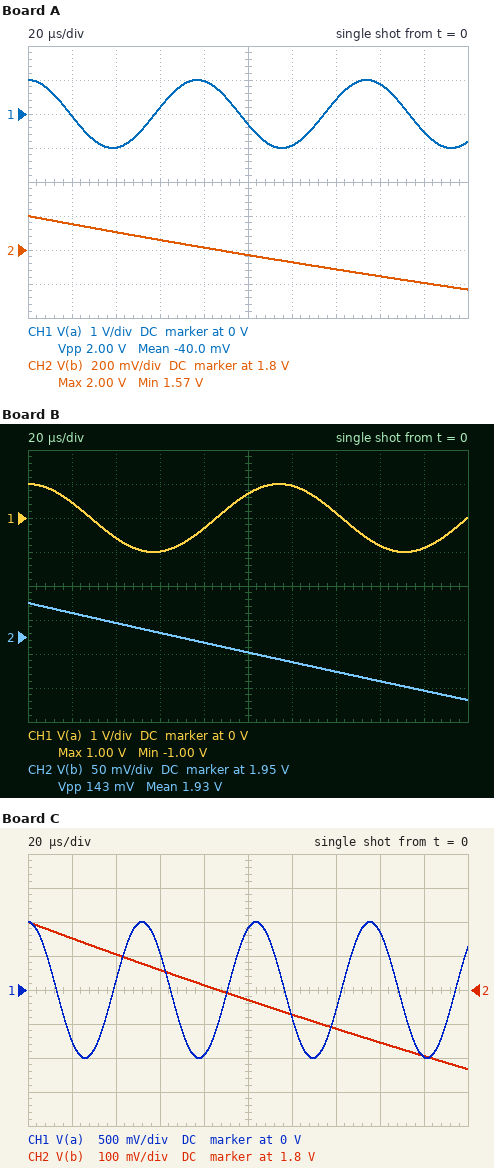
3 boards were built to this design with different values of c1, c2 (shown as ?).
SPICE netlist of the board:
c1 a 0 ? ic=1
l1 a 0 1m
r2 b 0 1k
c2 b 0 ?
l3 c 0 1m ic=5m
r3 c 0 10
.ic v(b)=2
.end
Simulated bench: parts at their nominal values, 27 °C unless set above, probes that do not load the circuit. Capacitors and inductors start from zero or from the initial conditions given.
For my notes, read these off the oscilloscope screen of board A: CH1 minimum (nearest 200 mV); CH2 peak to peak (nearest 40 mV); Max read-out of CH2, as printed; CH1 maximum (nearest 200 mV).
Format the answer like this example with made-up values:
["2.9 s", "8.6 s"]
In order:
["-1.0 V", "440 mV", "2.00 V", "1.0 V"]
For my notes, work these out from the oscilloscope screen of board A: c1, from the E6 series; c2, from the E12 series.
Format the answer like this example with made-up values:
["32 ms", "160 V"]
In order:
["150 nF", "820 nF"]
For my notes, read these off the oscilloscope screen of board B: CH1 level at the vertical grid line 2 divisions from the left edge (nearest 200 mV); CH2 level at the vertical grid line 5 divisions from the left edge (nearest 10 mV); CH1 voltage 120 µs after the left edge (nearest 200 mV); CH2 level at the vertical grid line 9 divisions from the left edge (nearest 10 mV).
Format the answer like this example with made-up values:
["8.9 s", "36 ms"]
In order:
["-600 mV", "1.93 V", "1.0 V", "1.87 V"]
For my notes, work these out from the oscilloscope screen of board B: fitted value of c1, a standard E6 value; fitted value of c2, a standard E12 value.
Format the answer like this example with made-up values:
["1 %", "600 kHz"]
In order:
["330 nF", "2.7 µF"]
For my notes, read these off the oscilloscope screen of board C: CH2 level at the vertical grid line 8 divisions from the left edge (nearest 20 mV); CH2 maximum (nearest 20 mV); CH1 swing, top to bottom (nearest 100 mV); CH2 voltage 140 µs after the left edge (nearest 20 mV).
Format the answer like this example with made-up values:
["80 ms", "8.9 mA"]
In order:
["1.64 V", "2.00 V", "2.0 V", "1.68 V"]
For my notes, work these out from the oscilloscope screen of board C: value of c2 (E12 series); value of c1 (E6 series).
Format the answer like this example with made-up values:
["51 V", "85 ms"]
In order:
["820 nF", "68 nF"]
